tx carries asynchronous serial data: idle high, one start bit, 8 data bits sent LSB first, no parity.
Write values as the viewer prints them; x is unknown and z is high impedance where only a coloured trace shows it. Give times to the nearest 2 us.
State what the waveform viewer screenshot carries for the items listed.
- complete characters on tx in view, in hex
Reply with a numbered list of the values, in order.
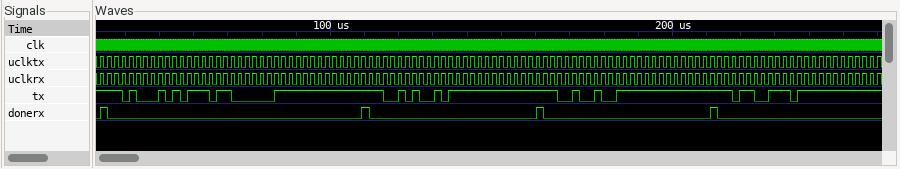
1. 51, 03, 4A, 92, 73
